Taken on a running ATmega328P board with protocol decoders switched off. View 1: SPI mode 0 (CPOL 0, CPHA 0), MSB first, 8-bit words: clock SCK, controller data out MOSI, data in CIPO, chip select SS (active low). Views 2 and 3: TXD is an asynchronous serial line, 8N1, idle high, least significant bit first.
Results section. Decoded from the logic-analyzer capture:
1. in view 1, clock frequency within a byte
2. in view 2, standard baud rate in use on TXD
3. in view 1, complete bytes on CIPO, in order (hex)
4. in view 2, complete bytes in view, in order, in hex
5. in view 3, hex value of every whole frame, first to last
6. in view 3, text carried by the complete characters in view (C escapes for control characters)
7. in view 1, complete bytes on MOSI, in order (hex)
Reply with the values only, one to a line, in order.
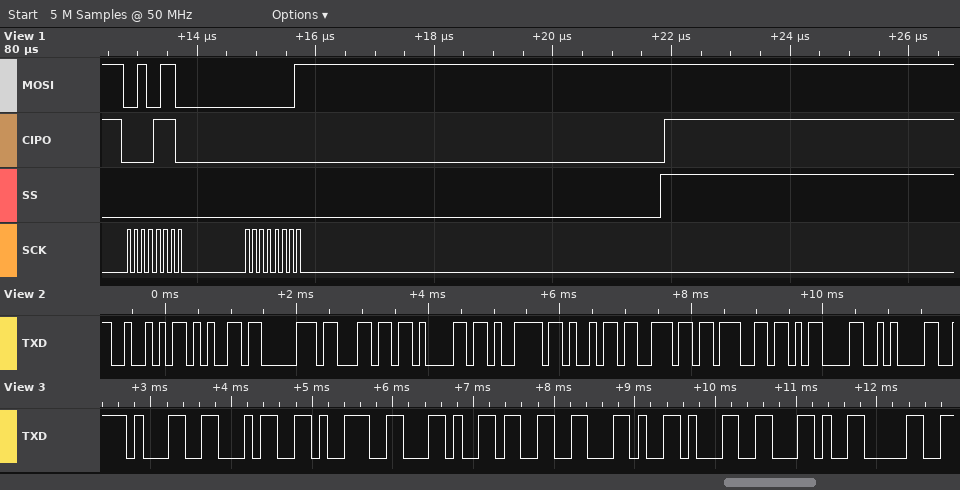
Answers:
8 MHz
9600 baud
0E 00
52 65 70 6C 61 79 69 6E 67 0D 0A
31 34 39 2C 33 2C 31 2C 30
"149,3,1,0"
26 01
